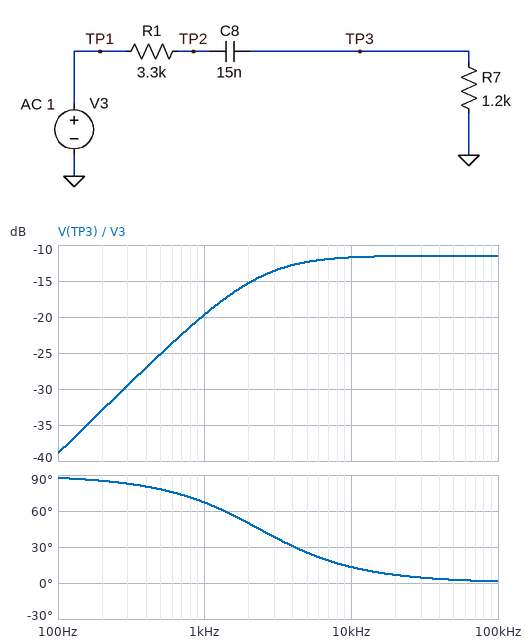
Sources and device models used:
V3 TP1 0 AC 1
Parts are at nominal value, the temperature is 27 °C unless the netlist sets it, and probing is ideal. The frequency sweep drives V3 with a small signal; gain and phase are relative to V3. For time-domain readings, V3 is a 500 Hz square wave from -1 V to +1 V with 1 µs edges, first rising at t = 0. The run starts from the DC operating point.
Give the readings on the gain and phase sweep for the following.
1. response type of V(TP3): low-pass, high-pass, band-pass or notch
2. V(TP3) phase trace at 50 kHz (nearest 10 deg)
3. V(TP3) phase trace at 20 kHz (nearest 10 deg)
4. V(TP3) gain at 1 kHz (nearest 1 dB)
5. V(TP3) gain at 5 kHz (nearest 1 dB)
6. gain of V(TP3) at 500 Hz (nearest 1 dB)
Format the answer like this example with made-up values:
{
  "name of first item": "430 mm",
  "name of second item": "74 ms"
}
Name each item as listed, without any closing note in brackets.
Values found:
{
  "response type of V(TP3): low-pass, high-pass, band-pass or notch": "high-pass",
  "V(TP3) phase trace at 50 kHz": "0 deg",
  "V(TP3) phase trace at 20 kHz": "10 deg",
  "V(TP3) gain at 1 kHz": "-20 dB",
  "V(TP3) gain at 5 kHz": "-12 dB",
  "gain of V(TP3) at 500 Hz": "-25 dB"
}
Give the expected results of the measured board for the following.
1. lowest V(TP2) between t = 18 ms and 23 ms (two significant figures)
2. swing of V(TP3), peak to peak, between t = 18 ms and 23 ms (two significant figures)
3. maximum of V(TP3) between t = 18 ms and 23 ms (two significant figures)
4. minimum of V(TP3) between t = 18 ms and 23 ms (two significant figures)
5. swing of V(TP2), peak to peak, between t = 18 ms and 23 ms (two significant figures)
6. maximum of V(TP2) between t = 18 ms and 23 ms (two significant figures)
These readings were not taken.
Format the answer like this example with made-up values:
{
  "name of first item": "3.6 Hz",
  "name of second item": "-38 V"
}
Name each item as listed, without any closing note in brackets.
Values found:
{
  "lowest V(TP2) between t = 18 ms and 23 ms": "-1.0 V",
  "swing of V(TP3), peak to peak, between t = 18 ms and 23 ms": "1.1 V",
  "maximum of V(TP3) between t = 18 ms and 23 ms": "530 mV",
  "minimum of V(TP3) between t = 18 ms and 23 ms": "-530 mV",
  "swing of V(TP2), peak to peak, between t = 18 ms and 23 ms": "2.0 V",
  "maximum of V(TP2) between t = 18 ms and 23 ms": "1.0 V"
}
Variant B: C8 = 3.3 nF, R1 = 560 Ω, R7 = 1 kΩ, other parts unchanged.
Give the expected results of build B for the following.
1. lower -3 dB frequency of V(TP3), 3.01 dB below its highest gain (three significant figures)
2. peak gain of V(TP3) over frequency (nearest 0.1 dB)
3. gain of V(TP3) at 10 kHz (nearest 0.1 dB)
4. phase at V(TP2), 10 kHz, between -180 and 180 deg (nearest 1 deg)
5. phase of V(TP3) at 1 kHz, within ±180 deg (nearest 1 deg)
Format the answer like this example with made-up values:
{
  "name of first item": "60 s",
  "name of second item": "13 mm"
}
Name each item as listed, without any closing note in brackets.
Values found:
{
  "lower -3 dB frequency of V(TP3), 3.01 dB below its highest gain": "30.9 kHz",
  "peak gain of V(TP3) over frequency": "-3.9 dB",
  "gain of V(TP3) at 10 kHz": "-14.1 dB",
  "phase at V(TP2), 10 kHz, between -180 and 180 deg": "-6 deg",
  "phase of V(TP3) at 1 kHz, within ±180 deg": "88 deg"
}
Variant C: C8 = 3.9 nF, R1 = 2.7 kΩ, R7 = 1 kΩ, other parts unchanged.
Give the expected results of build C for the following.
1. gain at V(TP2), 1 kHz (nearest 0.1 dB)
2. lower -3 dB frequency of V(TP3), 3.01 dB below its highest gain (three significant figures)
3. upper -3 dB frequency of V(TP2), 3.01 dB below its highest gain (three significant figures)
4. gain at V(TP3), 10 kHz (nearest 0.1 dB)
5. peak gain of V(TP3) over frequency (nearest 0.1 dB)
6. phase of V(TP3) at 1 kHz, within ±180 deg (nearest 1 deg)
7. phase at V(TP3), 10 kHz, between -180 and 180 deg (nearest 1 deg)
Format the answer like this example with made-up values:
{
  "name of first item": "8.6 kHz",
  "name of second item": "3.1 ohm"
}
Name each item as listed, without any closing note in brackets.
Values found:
{
  "gain at V(TP2), 1 kHz": "0 dB",
  "lower -3 dB frequency of V(TP3), 3.01 dB below its highest gain": "11.0 kHz",
  "upper -3 dB frequency of V(TP2), 3.01 dB below its highest gain": "11.9 kHz",
  "gain at V(TP3), 10 kHz": "-14.8 dB",
  "peak gain of V(TP3) over frequency": "-11.4 dB",
  "phase of V(TP3) at 1 kHz, within ±180 deg": "85 deg",
  "phase at V(TP3), 10 kHz, between -180 and 180 deg": "48 deg"
}
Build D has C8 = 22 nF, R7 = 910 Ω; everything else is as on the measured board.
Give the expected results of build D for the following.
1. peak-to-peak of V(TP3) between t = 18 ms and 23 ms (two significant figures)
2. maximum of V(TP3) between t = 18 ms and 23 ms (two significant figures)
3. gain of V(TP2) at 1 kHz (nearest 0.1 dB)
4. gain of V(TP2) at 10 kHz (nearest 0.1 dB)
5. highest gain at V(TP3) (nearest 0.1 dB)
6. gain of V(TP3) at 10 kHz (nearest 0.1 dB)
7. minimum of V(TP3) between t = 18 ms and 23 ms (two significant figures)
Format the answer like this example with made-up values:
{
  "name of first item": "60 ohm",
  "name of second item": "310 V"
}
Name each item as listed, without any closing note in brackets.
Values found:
{
  "peak-to-peak of V(TP3) between t = 18 ms and 23 ms": "860 mV",
  "maximum of V(TP3) between t = 18 ms and 23 ms": "430 mV",
  "gain of V(TP2) at 1 kHz": "-1.2 dB",
  "gain of V(TP2) at 10 kHz": "-11.3 dB",
  "highest gain at V(TP3)": "-13.3 dB",
  "gain of V(TP3) at 10 kHz": "-13.4 dB",
  "minimum of V(TP3) between t = 18 ms and 23 ms": "-430 mV"
}
